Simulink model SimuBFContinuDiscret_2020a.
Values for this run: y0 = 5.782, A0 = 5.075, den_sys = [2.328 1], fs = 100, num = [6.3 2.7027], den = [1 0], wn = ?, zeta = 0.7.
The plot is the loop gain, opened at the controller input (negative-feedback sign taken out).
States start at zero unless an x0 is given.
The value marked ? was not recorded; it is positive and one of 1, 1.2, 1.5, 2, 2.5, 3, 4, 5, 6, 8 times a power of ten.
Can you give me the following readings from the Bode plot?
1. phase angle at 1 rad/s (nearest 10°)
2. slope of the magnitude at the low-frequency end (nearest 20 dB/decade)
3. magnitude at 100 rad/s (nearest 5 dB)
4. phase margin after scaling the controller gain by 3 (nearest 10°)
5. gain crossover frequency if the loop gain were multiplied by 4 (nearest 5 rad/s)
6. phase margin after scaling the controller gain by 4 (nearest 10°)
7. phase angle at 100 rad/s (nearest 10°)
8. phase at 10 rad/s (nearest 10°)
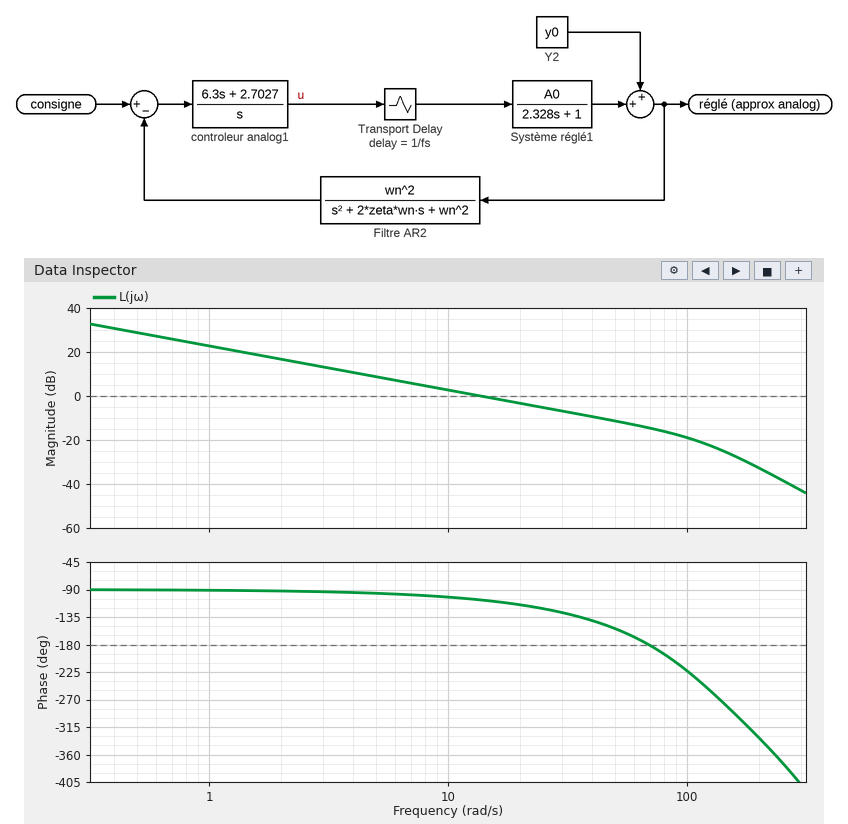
-90°
-20 dB/decade
-20 dB
40°
55 rad/s
20°
-220°
-100°
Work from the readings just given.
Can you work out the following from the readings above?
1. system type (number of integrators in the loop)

1
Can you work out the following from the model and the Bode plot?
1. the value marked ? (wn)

120
